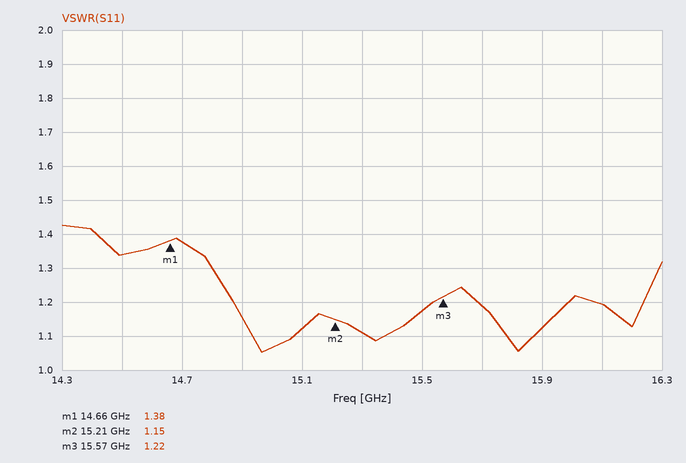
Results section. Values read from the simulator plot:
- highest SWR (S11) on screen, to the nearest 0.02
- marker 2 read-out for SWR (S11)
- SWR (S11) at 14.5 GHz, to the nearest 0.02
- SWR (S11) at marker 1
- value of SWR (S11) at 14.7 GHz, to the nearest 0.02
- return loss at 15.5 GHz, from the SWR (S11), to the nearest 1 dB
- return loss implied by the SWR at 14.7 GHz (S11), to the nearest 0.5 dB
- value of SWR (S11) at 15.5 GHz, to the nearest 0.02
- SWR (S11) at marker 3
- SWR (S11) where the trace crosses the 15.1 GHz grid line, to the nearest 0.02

1.42
1.15
1.34
1.38
1.38
22 dB
16.0 dB
1.18
1.22
1.12
